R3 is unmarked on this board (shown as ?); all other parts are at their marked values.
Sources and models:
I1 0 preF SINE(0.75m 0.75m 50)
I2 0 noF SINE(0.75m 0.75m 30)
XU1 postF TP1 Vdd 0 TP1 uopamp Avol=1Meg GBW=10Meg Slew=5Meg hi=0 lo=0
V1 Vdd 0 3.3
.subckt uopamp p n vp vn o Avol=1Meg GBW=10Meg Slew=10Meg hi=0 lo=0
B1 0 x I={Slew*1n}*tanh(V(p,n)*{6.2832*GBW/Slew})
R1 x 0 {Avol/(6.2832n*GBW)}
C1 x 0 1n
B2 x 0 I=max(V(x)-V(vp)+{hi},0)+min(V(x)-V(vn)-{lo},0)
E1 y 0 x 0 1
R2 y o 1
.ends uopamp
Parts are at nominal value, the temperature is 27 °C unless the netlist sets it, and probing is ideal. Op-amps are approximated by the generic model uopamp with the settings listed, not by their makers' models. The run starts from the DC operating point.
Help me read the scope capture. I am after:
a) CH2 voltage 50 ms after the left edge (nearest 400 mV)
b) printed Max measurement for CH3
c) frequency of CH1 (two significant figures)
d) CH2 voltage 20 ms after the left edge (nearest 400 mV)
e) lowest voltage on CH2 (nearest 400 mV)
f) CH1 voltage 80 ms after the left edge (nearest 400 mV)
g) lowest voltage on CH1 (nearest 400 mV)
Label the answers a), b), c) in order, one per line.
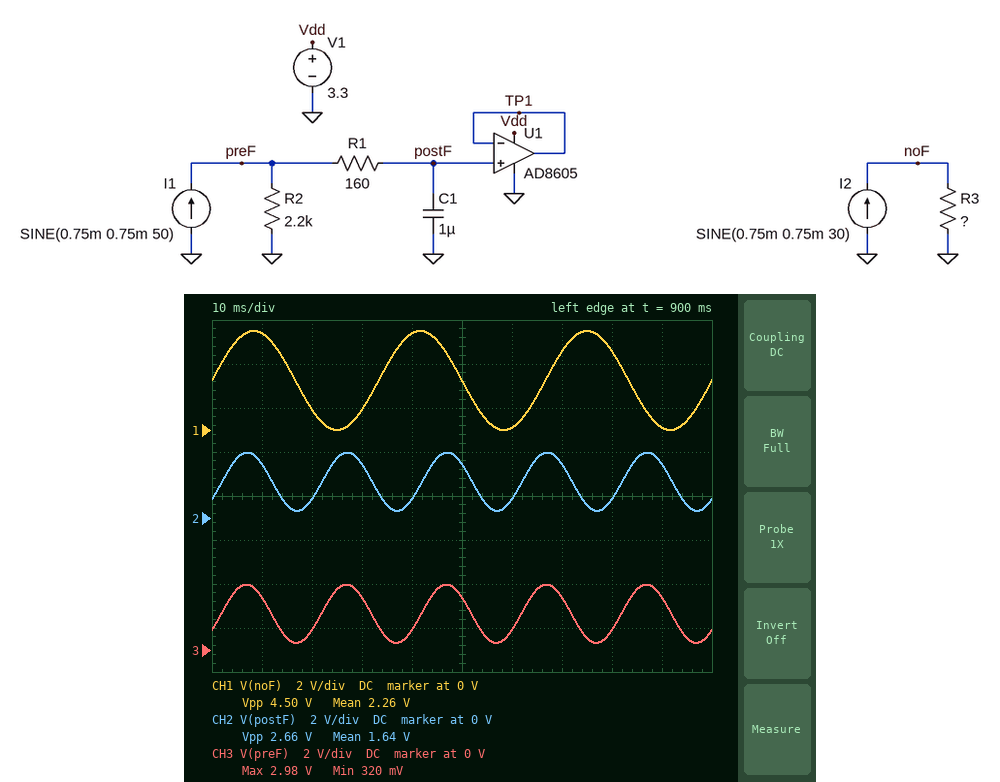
a) 2.4 V
b) 2.98 V
c) 30 Hz
d) 800 mV
e) 400 mV
f) 3.6 V
g) 0 V
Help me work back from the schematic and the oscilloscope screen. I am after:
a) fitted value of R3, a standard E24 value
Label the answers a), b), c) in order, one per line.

a) 3 kΩ
